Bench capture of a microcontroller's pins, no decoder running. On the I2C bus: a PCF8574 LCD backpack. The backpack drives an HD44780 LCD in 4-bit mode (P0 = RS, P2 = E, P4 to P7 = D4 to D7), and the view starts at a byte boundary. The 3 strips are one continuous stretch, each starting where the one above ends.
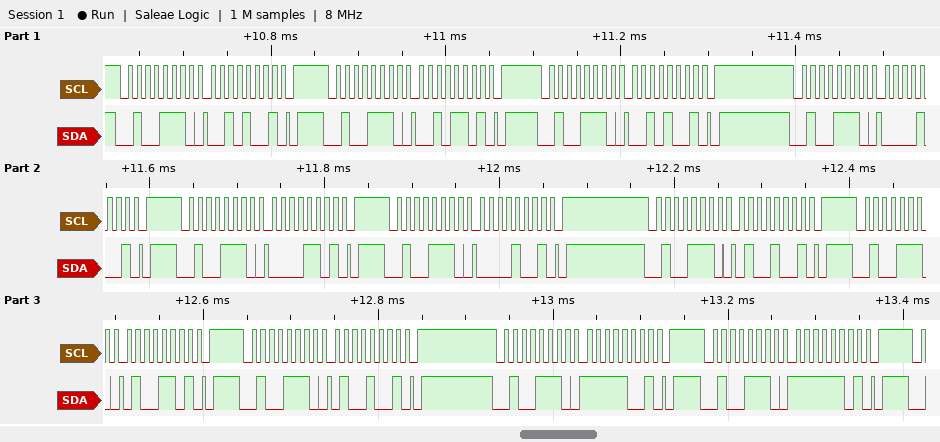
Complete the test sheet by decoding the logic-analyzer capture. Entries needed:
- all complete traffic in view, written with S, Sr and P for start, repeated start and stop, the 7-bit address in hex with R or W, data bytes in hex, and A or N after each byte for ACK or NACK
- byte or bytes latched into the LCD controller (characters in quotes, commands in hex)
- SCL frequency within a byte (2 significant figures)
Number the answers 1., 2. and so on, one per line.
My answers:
1. S 27W A 29 A P S 27W A 2D A P S 27W A 29 A P S 27W A 09 A P S 27W A 0D A P S 27W A 09 A P S 27W A 49 A P S 27W A 4D A P S 27W A 49 A P S 27W A F9 A P S 27W A FD A P
2. ' '
3. 100 kHz
